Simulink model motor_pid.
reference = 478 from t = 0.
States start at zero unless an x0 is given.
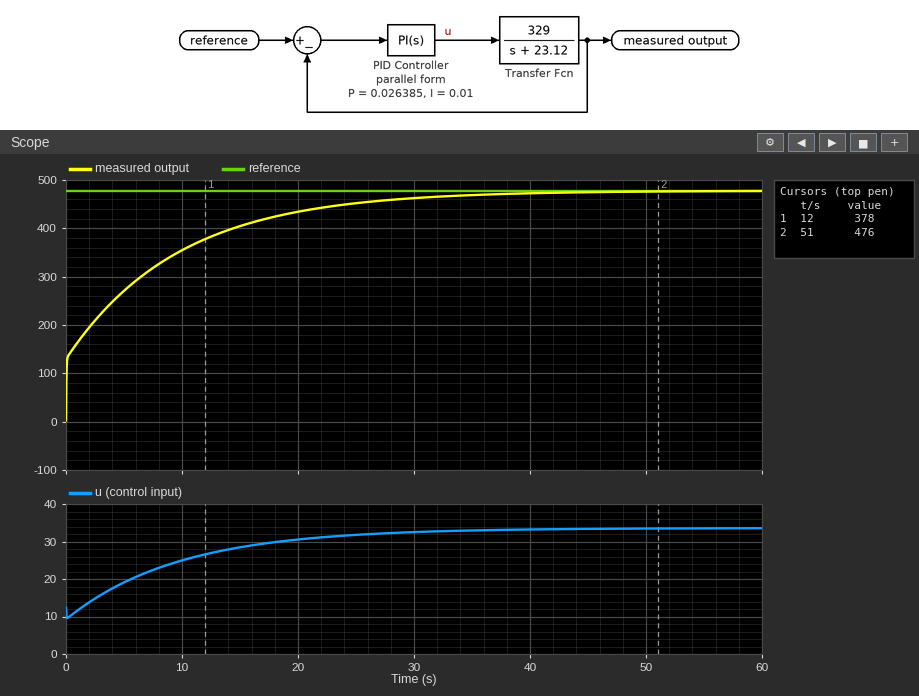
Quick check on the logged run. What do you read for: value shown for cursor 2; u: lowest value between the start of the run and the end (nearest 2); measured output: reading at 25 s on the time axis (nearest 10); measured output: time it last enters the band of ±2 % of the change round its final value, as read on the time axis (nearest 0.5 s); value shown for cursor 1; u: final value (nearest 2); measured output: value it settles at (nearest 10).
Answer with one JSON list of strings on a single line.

["476", "10", "450", "34.5 s", "378", "34", "480"]
